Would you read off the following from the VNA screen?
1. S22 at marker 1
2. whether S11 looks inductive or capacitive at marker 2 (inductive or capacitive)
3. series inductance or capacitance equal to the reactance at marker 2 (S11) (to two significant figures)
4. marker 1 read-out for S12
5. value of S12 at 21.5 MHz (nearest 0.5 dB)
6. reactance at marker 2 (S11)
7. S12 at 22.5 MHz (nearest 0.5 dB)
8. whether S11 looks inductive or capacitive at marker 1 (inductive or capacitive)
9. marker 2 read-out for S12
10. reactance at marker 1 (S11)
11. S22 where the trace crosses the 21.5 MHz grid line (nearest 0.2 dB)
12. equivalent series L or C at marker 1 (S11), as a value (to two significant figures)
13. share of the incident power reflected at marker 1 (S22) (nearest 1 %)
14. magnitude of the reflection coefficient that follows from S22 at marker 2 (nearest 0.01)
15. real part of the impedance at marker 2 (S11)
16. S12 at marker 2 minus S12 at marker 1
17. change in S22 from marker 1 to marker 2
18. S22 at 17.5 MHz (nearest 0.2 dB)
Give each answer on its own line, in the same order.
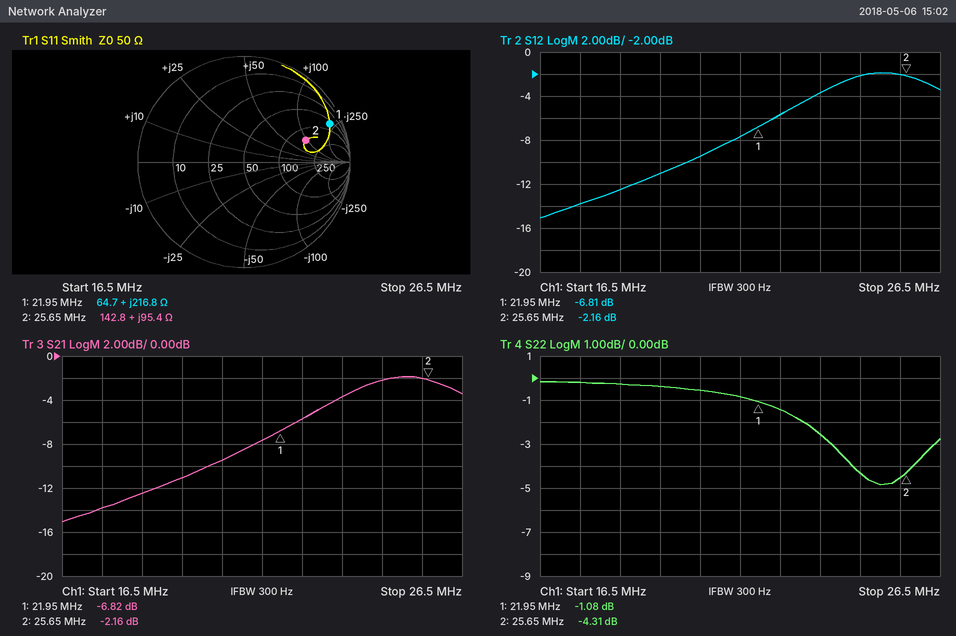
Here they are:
-1.08 dB
inductive
590 nH
-6.81 dB
-7.5 dB
+95.4 Ω
-5.5 dB
inductive
-2.16 dB
+216.8 Ω
-0.8 dB
1.6 µH
78 %
0.61
142.8 Ω
4.65 dB
-3.23 dB
-0.2 dB
